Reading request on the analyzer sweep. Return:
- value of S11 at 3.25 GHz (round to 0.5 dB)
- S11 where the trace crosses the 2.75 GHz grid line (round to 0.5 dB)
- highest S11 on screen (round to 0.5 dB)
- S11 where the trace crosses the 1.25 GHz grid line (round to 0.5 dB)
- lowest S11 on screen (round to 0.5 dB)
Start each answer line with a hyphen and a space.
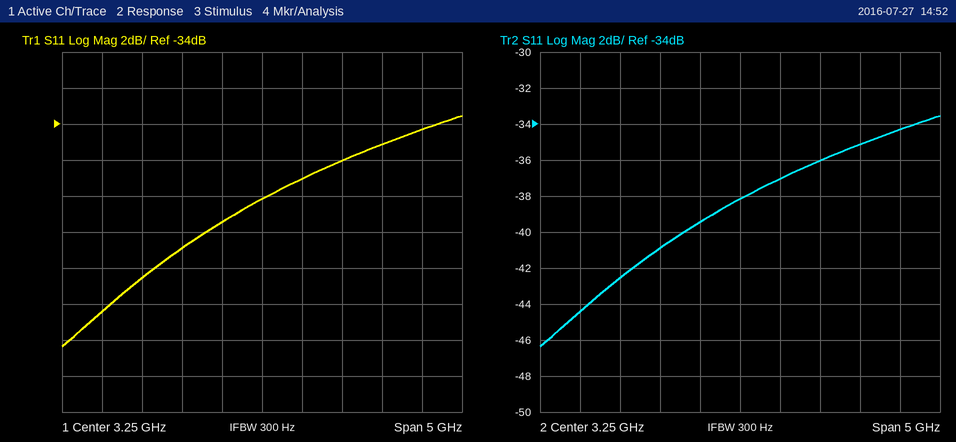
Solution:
- -38.0 dB
- -39.5 dB
- -33.5 dB
- -44.5 dB
- -46.5 dB
